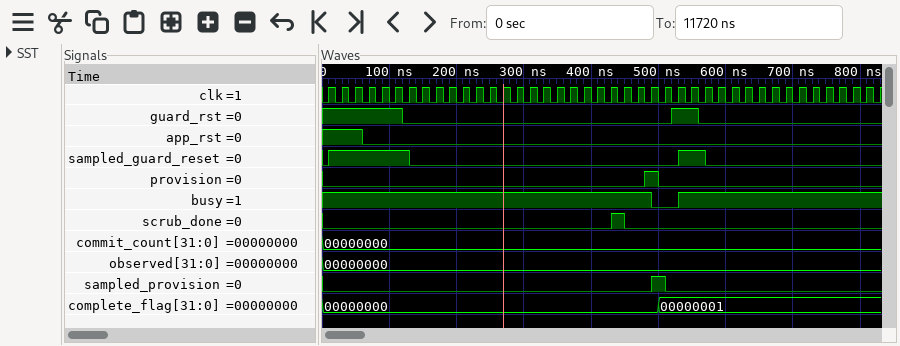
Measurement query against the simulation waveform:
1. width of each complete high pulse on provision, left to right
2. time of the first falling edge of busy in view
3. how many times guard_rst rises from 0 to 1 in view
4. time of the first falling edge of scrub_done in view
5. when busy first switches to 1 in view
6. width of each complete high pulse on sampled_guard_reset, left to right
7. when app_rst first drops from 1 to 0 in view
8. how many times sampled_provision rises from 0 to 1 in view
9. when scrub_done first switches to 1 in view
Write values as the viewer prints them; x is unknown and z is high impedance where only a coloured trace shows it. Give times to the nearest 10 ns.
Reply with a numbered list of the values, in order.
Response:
1. 20 ns
2. 490 ns
3. 1
4. 450 ns
5. 530 ns
6. 120 ns, 40 ns
7. 60 ns
8. 1
9. 430 ns
